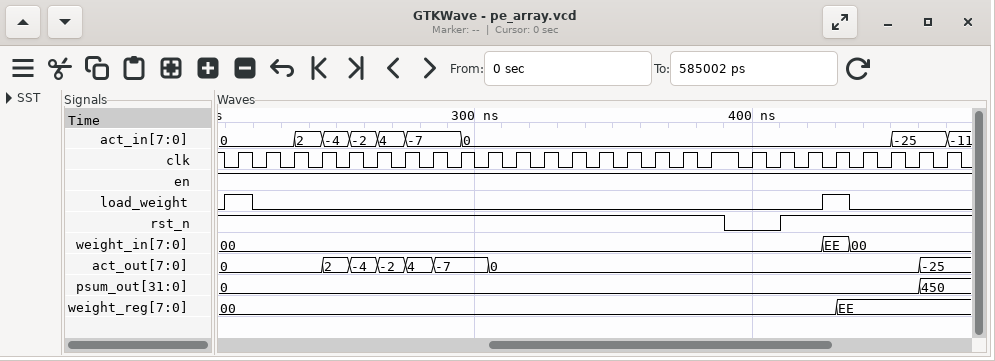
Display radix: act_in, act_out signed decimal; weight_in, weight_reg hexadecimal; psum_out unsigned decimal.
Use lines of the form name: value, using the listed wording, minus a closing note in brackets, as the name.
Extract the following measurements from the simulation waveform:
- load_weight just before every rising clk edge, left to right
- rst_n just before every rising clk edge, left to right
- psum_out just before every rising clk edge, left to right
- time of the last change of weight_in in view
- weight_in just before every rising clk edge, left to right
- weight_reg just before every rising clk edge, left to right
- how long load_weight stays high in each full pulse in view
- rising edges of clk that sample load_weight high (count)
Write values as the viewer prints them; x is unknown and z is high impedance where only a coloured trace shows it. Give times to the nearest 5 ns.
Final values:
load_weight just before every rising clk edge, left to right: 1 0 0 0 0 0 0 0 0 0 0 0 0 0 0 0 0 0 0 0 0 1 0 0 0 0
rst_n just before every rising clk edge, left to right: 1 1 1 1 1 1 1 1 1 1 1 1 1 1 1 1 1 1 0 0 1 1 1 1 1 1
psum_out just before every rising clk edge, left to right: 0, 0, 0, 0, 0, 0, 0, 0, 0, 0, 0, 0, 0, 0, 0, 0, 0, 0, 0, 0, 0, 0, 0, 0, 0, 450
time of the last change of weight_in in view: 435 ns
weight_in just before every rising clk edge, left to right: 00, 00, 00, 00, 00, 00, 00, 00, 00, 00, 00, 00, 00, 00, 00, 00, 00, 00, 00, 00, 00, EE, 00, 00, 00, 00
weight_reg just before every rising clk edge, left to right: 00, 00, 00, 00, 00, 00, 00, 00, 00, 00, 00, 00, 00, 00, 00, 00, 00, 00, 00, 00, 00, 00, EE, EE, EE, EE
how long load_weight stays high in each full pulse in view: 10 ns, 10 ns
rising edges of clk that sample load_weight high: 2
